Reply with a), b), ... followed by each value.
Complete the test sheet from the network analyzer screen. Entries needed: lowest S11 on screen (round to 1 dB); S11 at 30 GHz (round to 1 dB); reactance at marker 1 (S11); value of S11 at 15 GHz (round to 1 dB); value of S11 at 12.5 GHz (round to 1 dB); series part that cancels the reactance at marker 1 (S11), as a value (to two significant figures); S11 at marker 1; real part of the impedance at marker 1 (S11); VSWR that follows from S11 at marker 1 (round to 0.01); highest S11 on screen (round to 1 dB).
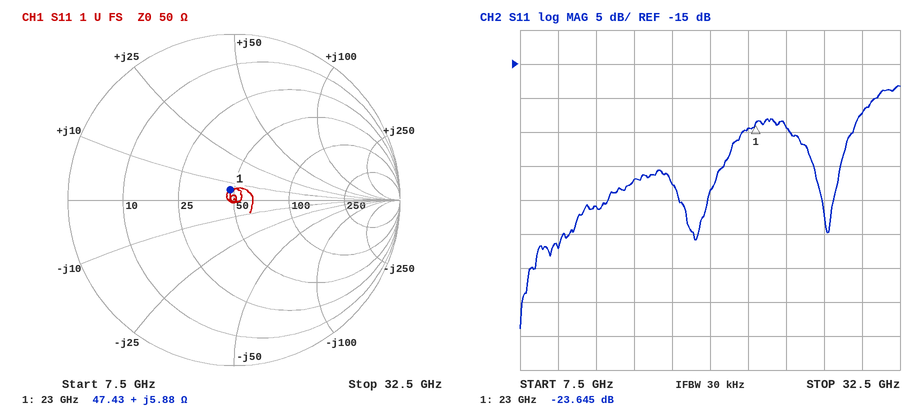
a) -54 dB
b) -22 dB
c) +5.88 Ω
d) -32 dB
e) -36 dB
f) 1.2 pF
g) -23.645 dB
h) 47.43 Ω
i) 1.14
j) -18 dB
